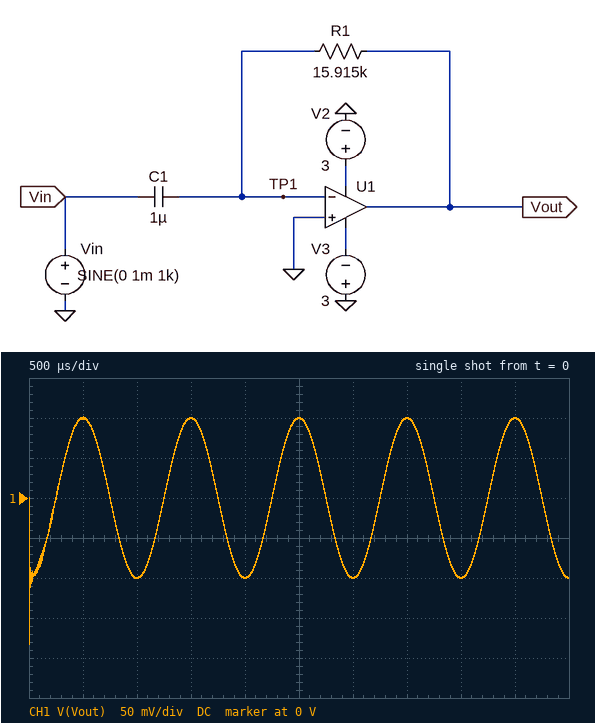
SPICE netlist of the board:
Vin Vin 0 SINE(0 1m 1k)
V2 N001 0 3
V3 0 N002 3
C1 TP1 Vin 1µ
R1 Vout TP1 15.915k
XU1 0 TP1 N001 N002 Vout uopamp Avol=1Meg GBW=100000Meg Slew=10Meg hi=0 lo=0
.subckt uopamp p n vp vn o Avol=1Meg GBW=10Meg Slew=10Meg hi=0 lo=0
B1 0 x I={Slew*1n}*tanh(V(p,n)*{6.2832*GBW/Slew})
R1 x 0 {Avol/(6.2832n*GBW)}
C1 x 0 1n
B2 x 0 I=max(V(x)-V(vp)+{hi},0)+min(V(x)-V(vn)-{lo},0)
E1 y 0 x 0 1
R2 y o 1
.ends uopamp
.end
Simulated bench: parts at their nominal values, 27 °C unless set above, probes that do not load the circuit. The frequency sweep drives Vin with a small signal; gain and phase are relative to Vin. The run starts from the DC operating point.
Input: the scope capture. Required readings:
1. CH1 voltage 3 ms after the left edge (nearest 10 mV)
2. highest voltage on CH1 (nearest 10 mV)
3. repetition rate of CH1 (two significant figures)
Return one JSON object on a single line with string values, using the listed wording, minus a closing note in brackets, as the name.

{"CH1 voltage 3 ms after the left edge": "-100 mV", "highest voltage on CH1": "100 mV", "repetition rate of CH1": "1.0 kHz"}
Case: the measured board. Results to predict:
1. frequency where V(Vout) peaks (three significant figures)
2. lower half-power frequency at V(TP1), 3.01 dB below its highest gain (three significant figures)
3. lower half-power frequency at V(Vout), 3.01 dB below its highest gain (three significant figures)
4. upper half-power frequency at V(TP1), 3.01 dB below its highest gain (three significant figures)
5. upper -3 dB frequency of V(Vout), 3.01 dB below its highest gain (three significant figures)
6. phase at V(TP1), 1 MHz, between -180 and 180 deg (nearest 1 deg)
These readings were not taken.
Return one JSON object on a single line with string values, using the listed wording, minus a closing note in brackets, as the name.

{"frequency where V(Vout) peaks": "1.00 MHz", "lower half-power frequency at V(TP1), 3.01 dB below its highest gain": "956 kHz", "lower half-power frequency at V(Vout), 3.01 dB below its highest gain": "951 kHz", "upper half-power frequency at V(TP1), 3.01 dB below its highest gain": "1.06 MHz", "upper -3 dB frequency of V(Vout), 3.01 dB below its highest gain": "1.05 MHz", "phase at V(TP1), 1 MHz, between -180 and 180 deg": "84 deg"}
